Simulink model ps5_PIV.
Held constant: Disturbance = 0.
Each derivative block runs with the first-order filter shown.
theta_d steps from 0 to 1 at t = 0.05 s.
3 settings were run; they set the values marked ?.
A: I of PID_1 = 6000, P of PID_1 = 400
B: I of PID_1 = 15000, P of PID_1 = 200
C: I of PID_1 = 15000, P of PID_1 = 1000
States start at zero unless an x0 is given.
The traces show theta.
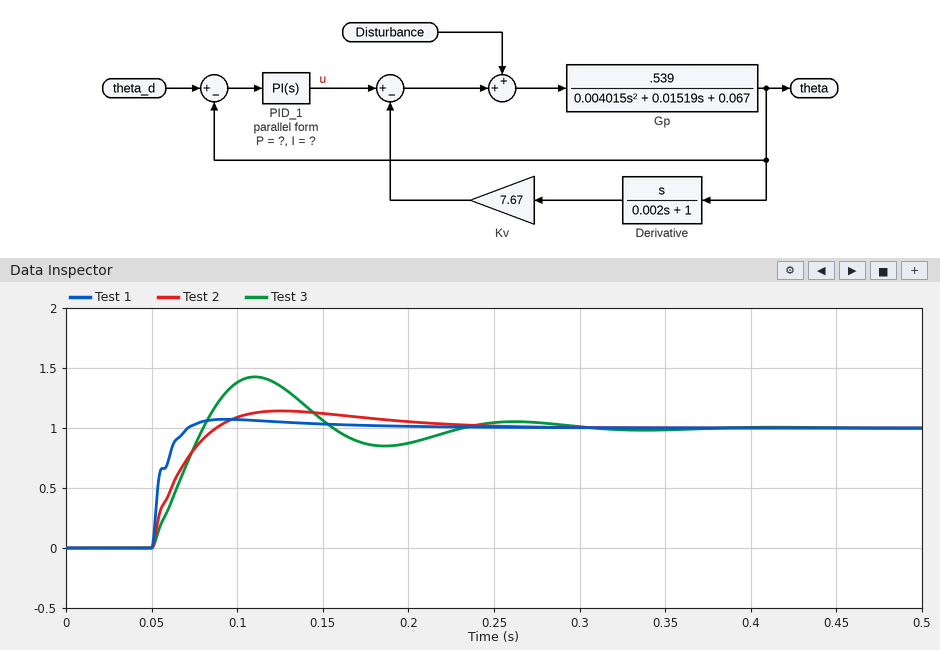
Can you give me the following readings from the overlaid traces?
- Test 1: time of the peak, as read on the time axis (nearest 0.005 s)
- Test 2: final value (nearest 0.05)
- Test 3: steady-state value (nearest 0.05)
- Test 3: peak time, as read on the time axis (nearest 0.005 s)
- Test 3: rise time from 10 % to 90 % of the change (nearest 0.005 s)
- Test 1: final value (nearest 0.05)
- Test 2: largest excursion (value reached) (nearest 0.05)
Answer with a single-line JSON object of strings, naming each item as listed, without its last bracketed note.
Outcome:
{"Test 1: time of the peak, as read on the time axis": "0.095 s", "Test 2: final value": "1.00", "Test 3: steady-state value": "1.00", "Test 3: peak time, as read on the time axis": "0.110 s", "Test 3: rise time from 10 % to 90 % of the change": "0.025 s", "Test 1: final value": "1.00", "Test 2: largest excursion (value reached)": "1.15"}
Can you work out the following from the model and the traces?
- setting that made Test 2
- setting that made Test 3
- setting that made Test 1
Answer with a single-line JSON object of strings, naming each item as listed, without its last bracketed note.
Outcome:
{"setting that made Test 2": "A", "setting that made Test 3": "B", "setting that made Test 1": "C"}
